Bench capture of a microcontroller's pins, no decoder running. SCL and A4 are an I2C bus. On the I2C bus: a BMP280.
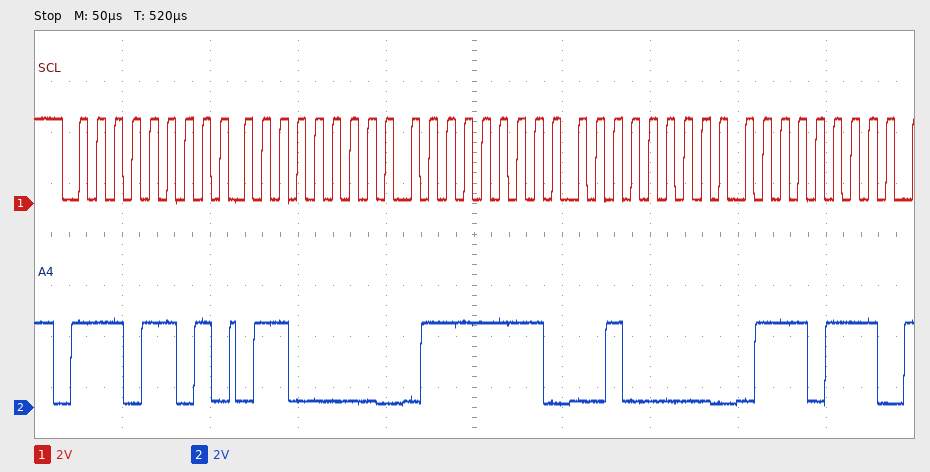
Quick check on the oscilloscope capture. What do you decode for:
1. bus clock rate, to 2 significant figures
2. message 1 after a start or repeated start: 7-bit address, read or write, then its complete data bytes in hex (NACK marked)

100 kHz
0x76 read: 60 7F 20 77
